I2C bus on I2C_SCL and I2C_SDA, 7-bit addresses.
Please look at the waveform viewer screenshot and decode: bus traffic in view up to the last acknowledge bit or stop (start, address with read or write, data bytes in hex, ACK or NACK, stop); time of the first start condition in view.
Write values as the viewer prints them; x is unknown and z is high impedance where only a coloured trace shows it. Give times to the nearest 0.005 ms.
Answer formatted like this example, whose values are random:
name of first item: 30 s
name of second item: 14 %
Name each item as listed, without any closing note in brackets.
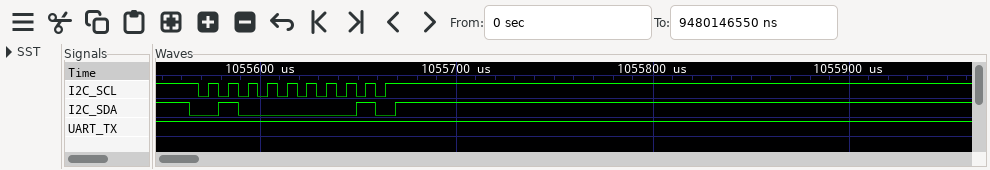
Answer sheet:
bus traffic in view up to the last acknowledge bit or stop: start, address 20 write NACK, stop
time of the first start condition in view: 1055.565 ms
